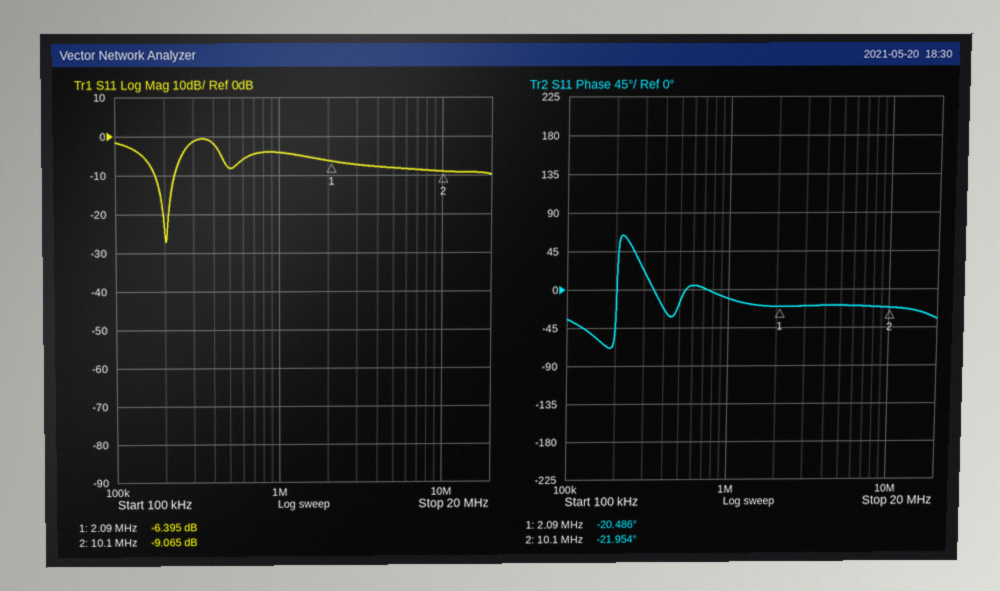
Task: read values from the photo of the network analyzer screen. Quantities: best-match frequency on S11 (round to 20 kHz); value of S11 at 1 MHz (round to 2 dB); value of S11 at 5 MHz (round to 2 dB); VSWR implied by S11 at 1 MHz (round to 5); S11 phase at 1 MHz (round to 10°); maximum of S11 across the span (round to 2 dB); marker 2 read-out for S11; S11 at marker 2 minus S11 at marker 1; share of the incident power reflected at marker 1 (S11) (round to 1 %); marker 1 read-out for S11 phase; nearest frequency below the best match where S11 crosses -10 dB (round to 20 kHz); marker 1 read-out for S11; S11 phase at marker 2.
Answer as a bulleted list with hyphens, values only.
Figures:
- 200 kHz
- -4 dB
- -8 dB
- 5
- -10°
- 0 dB
- -9.065 dB
- -2.670 dB
- 23 %
- -20.486°
- 180 kHz
- -6.395 dB
- -21.954°
